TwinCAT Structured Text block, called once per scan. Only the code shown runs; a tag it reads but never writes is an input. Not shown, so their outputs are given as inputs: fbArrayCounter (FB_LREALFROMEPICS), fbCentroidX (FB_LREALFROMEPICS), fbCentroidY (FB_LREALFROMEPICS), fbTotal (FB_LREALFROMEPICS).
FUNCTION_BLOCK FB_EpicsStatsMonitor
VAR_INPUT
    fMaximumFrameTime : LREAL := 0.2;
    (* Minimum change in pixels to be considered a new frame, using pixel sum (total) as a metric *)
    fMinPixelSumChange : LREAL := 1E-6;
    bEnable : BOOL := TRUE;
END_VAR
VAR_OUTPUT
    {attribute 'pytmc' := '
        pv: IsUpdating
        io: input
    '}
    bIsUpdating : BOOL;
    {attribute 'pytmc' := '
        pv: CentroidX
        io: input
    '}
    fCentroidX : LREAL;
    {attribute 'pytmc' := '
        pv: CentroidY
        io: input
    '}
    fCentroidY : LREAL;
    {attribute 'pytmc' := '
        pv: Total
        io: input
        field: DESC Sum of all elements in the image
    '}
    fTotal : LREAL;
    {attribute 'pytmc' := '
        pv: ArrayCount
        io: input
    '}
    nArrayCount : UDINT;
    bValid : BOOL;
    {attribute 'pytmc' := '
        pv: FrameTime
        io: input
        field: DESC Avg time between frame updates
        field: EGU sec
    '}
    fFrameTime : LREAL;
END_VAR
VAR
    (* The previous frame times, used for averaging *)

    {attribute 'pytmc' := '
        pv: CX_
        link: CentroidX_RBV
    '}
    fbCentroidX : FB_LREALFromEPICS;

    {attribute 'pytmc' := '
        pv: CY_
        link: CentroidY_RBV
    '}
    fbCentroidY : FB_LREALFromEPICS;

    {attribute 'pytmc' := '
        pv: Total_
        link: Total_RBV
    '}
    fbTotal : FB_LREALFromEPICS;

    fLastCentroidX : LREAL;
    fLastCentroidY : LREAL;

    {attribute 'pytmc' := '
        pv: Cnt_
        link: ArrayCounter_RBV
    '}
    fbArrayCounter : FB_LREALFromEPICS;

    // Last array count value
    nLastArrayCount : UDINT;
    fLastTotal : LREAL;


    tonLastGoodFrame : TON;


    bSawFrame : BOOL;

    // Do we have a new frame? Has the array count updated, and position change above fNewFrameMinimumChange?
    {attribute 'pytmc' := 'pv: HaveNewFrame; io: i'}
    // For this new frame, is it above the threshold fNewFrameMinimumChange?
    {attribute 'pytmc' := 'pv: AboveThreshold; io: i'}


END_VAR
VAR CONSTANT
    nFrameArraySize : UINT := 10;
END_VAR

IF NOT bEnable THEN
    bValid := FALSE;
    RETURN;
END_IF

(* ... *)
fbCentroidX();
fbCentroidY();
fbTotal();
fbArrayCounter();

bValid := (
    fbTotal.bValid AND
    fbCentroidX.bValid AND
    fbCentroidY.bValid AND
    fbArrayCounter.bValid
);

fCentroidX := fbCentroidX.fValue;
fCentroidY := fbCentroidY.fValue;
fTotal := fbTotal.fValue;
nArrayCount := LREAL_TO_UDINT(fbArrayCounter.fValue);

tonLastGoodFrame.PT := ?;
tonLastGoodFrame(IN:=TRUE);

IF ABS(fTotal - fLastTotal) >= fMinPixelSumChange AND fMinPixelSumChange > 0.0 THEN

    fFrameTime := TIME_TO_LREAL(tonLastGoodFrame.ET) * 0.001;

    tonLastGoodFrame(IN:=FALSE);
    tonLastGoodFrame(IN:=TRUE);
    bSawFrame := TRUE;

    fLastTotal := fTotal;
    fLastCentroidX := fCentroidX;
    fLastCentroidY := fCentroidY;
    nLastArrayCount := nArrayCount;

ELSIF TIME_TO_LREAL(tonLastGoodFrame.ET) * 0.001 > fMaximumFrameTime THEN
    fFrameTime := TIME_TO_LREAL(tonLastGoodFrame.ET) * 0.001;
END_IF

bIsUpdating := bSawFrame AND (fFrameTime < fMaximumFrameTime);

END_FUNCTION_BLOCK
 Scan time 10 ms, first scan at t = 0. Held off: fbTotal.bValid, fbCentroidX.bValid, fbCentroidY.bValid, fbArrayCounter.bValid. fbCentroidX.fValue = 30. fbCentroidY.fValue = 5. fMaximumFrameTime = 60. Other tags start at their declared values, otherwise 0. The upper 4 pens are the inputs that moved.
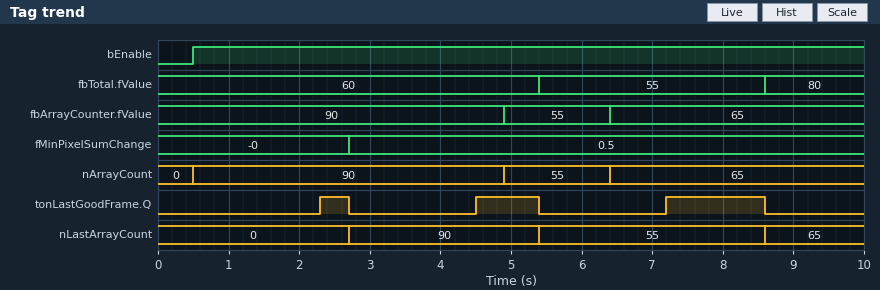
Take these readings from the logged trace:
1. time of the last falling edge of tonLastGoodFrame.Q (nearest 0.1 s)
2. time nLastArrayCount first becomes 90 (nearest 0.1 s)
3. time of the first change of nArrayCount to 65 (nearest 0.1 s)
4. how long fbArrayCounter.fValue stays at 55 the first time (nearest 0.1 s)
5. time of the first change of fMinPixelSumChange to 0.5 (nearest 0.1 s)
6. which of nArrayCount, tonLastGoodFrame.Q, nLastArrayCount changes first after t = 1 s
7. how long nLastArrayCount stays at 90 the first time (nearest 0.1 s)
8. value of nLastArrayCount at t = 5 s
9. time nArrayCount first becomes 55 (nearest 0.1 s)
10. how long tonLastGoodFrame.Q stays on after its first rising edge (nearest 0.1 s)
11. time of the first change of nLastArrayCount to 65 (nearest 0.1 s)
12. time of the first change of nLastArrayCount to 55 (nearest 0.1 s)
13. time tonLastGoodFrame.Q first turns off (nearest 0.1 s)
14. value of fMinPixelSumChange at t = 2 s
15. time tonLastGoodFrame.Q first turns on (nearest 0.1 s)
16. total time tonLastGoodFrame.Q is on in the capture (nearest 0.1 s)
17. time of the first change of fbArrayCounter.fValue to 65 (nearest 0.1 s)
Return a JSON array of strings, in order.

["8.6 s", "2.7 s", "6.4 s", "1.5 s", "2.7 s", "tonLastGoodFrame.Q", "2.7 s", "90", "4.9 s", "0.4 s", "8.6 s", "5.4 s", "2.7 s", "-0", "2.3 s", "2.7 s", "6.4 s"]
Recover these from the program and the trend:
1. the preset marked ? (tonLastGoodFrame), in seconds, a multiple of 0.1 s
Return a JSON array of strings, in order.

["1.8 s"]
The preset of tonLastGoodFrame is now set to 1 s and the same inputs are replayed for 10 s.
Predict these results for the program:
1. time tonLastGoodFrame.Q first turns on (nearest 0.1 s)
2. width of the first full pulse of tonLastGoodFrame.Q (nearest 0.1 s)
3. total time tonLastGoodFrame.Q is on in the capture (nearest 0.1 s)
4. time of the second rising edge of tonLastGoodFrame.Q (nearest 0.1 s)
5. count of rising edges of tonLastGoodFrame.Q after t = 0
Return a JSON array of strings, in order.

["1.5 s", "1.2 s", "5.5 s", "3.7 s", "4"]
